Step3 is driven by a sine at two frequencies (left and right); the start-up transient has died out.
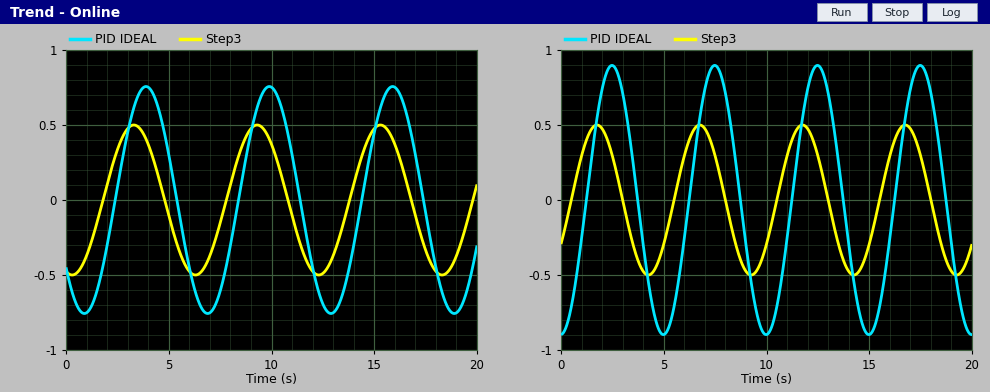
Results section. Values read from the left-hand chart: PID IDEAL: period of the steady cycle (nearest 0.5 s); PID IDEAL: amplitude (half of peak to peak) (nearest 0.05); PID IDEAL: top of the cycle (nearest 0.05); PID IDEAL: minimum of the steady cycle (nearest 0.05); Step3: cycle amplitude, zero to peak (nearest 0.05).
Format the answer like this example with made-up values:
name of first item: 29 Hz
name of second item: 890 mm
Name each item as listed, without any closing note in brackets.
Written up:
PID IDEAL: period of the steady cycle: 6.0 s
PID IDEAL: amplitude (half of peak to peak): 0.75
PID IDEAL: top of the cycle: 0.75
PID IDEAL: minimum of the steady cycle: -0.75
Step3: cycle amplitude, zero to peak: 0.50
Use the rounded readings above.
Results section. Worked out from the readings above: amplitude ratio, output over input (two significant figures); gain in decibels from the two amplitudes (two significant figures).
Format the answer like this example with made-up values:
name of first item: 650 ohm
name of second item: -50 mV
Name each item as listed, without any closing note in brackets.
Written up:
amplitude ratio, output over input: 1.5
gain in decibels from the two amplitudes: 3.5 dB
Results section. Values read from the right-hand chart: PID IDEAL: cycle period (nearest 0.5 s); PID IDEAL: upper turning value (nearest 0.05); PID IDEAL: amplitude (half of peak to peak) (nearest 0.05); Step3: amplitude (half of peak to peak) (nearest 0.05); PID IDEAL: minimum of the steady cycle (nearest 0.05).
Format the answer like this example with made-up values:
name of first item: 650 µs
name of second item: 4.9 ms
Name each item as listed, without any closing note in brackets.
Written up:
PID IDEAL: cycle period: 5.0 s
PID IDEAL: upper turning value: 0.90
PID IDEAL: amplitude (half of peak to peak): 0.90
Step3: amplitude (half of peak to peak): 0.50
PID IDEAL: minimum of the steady cycle: -0.90
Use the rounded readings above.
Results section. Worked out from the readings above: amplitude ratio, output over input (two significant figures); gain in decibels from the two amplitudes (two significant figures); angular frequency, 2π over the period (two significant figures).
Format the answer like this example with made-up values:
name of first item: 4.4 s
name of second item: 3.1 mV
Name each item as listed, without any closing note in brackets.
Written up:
amplitude ratio, output over input: 1.8
gain in decibels from the two amplitudes: 5.1 dB
angular frequency, 2π over the period: 1.3 rad/s
